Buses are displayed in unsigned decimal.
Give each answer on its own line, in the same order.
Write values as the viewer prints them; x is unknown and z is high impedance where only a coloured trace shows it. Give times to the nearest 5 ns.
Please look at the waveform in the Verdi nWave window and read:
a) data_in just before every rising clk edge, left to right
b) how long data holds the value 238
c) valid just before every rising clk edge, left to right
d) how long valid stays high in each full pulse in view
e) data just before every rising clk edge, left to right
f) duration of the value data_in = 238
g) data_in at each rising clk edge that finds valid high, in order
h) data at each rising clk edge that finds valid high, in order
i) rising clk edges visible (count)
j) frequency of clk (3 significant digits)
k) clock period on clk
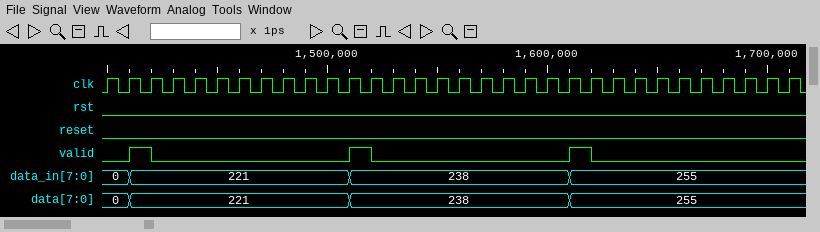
0, 0, 221, 221, 221, 221, 221, 221, 221, 221, 221, 221, 238, 238, 238, 238, 238, 238, 238, 238, 238, 238, 255, 255, 255, 255, 255, 255, 255, 255, 255, 255
100 ns
0 0 1 0 0 0 0 0 0 0 0 0 1 0 0 0 0 0 0 0 0 0 1 0 0 0 0 0 0 0 0 0
10 ns, 10 ns, 10 ns
0, 0, 221, 221, 221, 221, 221, 221, 221, 221, 221, 221, 238, 238, 238, 238, 238, 238, 238, 238, 238, 238, 255, 255, 255, 255, 255, 255, 255, 255, 255, 255
100 ns
221, 238, 255
221, 238, 255
32
100 MHz
10 ns
